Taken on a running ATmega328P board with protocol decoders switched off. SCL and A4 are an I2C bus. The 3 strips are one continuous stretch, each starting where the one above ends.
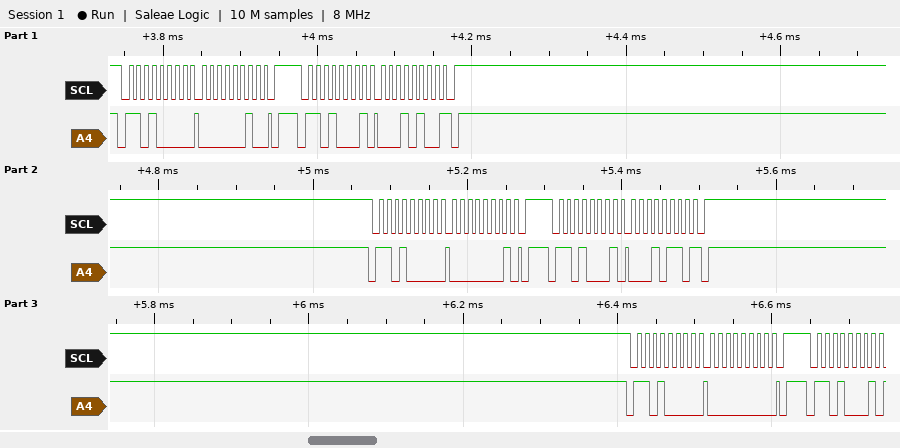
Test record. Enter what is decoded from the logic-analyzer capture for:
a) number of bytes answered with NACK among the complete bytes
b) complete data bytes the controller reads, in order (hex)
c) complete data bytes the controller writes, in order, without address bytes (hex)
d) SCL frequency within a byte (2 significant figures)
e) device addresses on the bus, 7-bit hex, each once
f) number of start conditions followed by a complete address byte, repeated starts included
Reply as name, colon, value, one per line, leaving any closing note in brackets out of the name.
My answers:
number of bytes answered with NACK among the complete bytes: 2
complete data bytes the controller reads, in order: 14 16
complete data bytes the controller writes, in order, without address bytes: 02 01 00
SCL frequency within a byte: 100 kHz
device addresses on the bus, 7-bit hex, each once: 0x68
number of start conditions followed by a complete address byte, repeated starts included: 6
